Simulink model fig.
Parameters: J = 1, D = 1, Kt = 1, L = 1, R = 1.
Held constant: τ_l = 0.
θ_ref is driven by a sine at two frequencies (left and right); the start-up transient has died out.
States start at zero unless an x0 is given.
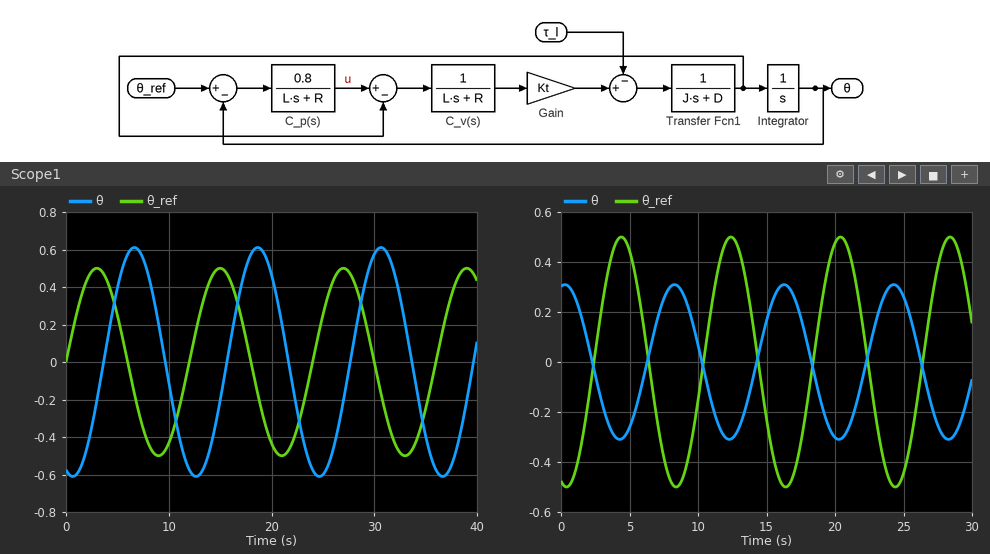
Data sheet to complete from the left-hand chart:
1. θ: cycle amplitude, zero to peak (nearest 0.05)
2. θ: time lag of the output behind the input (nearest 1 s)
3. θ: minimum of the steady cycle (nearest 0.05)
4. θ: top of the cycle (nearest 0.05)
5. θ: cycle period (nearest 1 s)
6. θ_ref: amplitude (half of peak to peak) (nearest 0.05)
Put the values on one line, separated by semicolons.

0.60; 4 s; -0.60; 0.60; 12 s; 0.50
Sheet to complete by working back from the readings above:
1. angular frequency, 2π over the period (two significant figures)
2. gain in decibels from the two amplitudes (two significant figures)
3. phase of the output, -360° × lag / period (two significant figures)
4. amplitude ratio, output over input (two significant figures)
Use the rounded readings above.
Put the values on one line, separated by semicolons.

0.52 rad/s; 1.6 dB; -120°; 1.2
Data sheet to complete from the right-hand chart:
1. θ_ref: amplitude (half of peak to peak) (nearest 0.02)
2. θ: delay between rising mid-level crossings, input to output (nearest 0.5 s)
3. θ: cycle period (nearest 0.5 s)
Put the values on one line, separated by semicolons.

0.50; 4.0 s; 8.0 s
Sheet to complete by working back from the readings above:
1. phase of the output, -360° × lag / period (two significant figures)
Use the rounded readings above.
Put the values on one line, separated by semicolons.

-180°
